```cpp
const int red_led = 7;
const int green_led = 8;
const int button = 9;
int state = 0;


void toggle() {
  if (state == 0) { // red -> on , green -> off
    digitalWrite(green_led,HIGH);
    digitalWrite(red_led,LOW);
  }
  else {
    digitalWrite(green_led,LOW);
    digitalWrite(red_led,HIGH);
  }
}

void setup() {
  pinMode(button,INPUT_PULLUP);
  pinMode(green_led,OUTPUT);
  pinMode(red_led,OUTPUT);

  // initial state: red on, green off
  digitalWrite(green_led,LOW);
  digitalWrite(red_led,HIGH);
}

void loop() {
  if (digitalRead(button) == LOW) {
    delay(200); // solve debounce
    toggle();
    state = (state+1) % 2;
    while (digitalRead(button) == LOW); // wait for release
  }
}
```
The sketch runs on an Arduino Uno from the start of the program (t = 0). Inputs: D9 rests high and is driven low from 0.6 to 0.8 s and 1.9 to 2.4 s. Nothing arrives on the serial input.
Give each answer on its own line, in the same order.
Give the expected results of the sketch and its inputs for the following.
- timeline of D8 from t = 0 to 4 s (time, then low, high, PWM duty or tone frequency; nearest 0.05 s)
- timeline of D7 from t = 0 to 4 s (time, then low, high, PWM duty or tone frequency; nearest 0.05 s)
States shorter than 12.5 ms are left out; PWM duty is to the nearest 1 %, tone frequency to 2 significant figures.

0 s low; 0.8 s high; 2.1 s low
0 s high; 0.8 s low; 2.1 s high
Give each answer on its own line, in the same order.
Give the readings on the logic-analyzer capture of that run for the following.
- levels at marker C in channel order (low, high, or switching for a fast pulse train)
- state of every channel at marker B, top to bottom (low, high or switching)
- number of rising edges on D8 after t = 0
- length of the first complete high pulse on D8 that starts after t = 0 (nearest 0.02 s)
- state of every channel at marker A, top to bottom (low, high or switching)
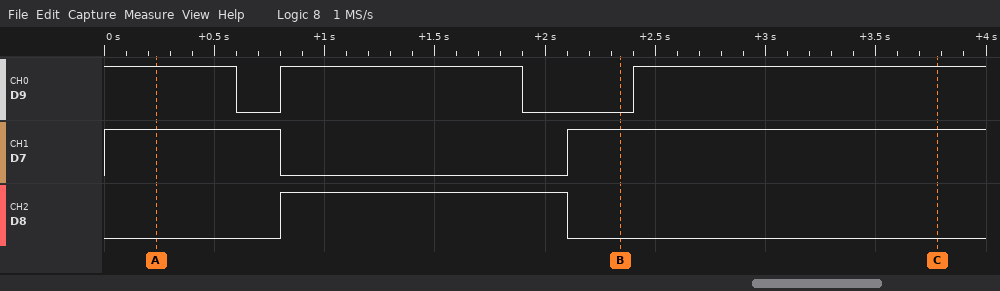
D9 high, D7 high, D8 low
D9 low, D7 high, D8 low
1
1.30 s
D9 high, D7 high, D8 low
